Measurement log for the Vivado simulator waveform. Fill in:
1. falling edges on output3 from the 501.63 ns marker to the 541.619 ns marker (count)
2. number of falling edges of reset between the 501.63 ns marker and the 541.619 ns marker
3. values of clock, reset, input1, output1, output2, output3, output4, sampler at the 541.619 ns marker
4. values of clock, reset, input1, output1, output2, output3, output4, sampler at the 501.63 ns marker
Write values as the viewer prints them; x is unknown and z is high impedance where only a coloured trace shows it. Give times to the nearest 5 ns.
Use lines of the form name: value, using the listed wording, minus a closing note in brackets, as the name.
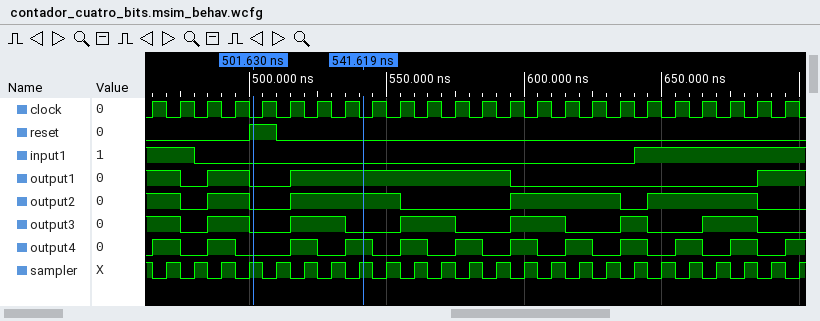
falling edges on output3 from the 501.63 ns marker to the 541.619 ns marker: 1
number of falling edges of reset between the 501.63 ns marker and the 541.619 ns marker: 1
values of clock, reset, input1, output1, output2, output3, output4, sampler at the 541.619 ns marker: clock=0, reset=0, input1=0, output1=1, output2=1, output3=0, output4=1, sampler=1
values of clock, reset, input1, output1, output2, output3, output4, sampler at the 501.63 ns marker: clock=0, reset=1, input1=0, output1=0, output2=0, output3=0, output4=0, sampler=1
